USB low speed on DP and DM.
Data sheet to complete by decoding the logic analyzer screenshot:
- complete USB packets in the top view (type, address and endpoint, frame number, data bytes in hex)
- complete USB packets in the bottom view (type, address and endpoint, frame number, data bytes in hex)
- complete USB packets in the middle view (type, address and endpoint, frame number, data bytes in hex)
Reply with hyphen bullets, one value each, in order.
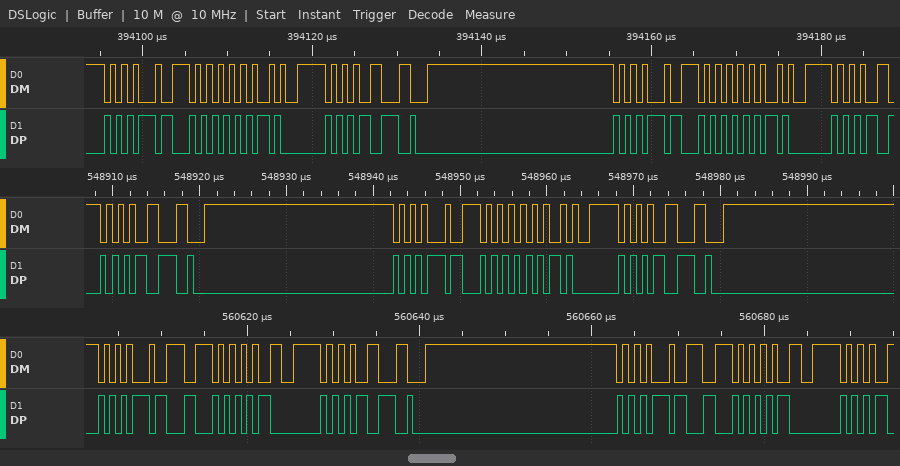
- IN ADDR 0 EP 0, NAK, IN ADDR 0 EP 0
- IN ADDR 13 EP 0, NAK, IN ADDR 13 EP 0
- NAK, IN ADDR 0 EP 0, NAK
